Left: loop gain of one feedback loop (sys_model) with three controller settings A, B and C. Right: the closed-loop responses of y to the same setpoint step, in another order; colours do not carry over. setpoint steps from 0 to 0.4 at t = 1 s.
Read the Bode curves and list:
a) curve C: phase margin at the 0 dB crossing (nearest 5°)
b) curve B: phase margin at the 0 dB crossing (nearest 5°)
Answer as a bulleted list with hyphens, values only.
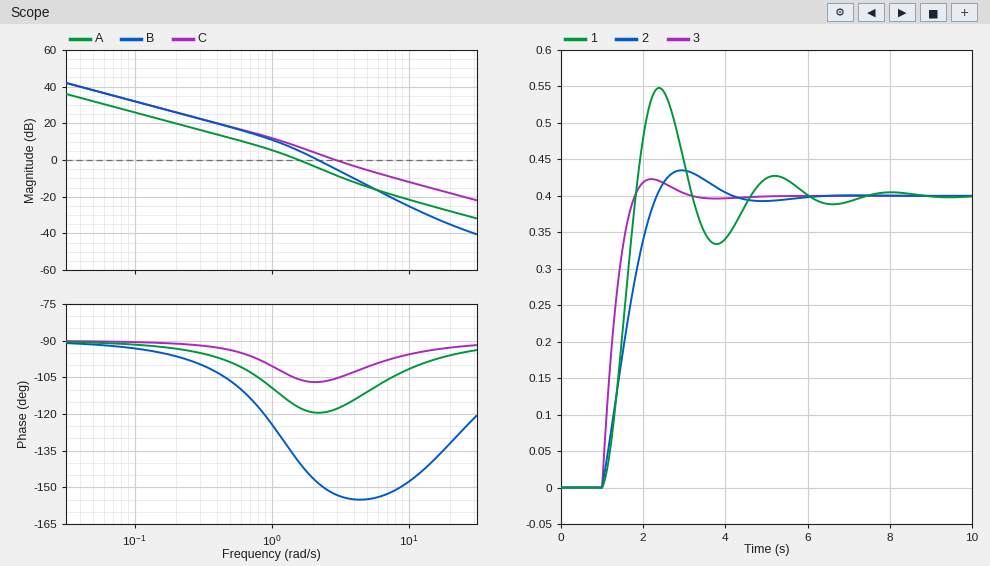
- 75°
- 30°
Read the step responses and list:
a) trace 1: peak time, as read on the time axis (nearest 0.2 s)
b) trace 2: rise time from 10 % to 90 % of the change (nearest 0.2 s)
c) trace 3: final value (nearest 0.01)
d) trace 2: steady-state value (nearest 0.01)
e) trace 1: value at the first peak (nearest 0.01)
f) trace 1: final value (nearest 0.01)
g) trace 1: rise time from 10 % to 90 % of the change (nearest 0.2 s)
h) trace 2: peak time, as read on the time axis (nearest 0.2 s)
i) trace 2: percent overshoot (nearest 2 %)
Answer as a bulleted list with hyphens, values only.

- 2.4 s
- 1.0 s
- 0.40
- 0.40
- 0.55
- 0.40
- 0.6 s
- 3.0 s
- 8 %
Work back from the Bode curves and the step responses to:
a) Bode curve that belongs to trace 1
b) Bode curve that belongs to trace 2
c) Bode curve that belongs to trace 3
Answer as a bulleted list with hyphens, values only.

- B
- A
- C
